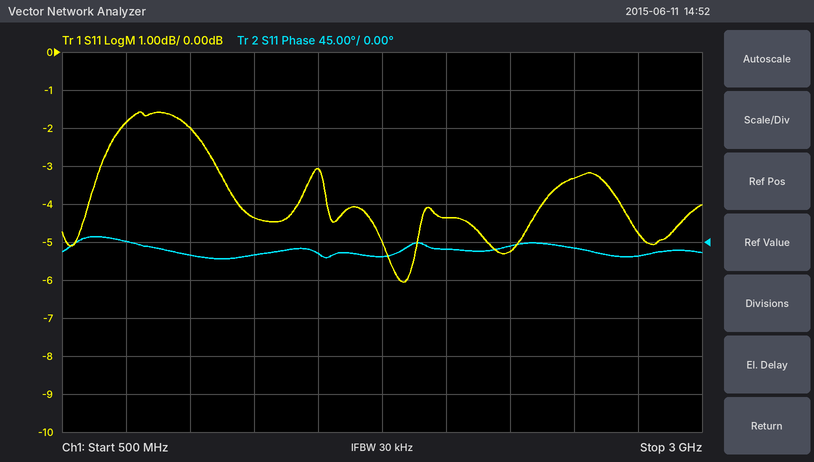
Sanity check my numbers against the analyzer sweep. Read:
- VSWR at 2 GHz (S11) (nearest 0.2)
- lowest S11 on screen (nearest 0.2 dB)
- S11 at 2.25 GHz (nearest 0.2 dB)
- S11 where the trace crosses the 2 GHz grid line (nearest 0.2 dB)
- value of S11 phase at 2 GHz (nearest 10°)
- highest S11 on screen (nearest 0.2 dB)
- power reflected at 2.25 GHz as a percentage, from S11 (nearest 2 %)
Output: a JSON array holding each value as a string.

["4.0", "-6.0 dB", "-5.2 dB", "-4.4 dB", "-10°", "-1.6 dB", "30 %"]
